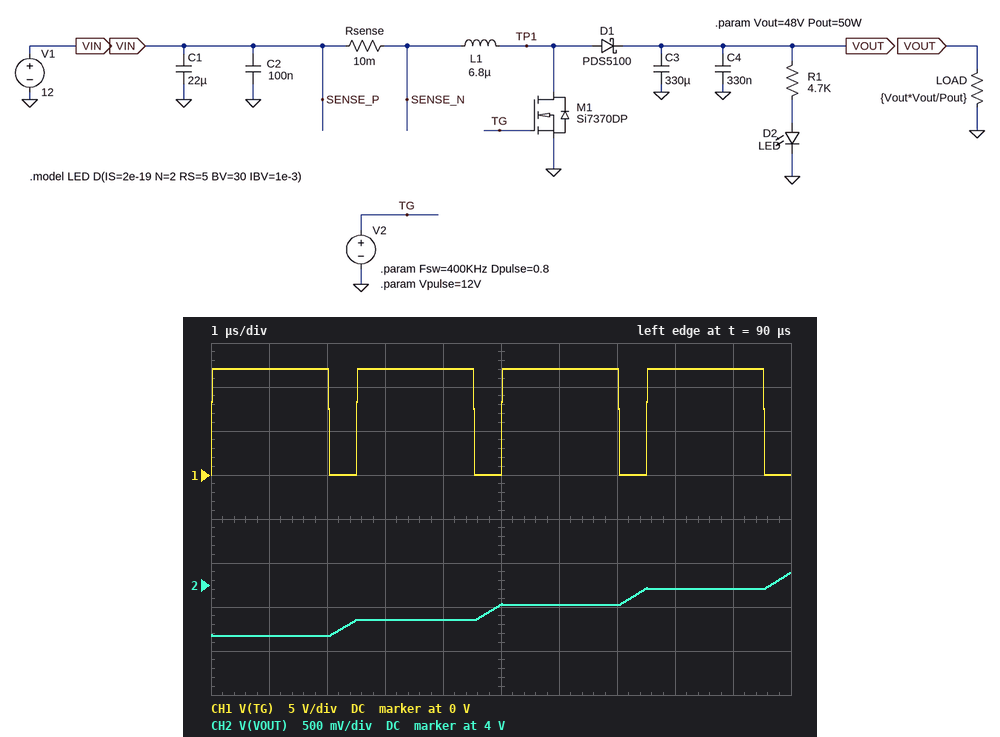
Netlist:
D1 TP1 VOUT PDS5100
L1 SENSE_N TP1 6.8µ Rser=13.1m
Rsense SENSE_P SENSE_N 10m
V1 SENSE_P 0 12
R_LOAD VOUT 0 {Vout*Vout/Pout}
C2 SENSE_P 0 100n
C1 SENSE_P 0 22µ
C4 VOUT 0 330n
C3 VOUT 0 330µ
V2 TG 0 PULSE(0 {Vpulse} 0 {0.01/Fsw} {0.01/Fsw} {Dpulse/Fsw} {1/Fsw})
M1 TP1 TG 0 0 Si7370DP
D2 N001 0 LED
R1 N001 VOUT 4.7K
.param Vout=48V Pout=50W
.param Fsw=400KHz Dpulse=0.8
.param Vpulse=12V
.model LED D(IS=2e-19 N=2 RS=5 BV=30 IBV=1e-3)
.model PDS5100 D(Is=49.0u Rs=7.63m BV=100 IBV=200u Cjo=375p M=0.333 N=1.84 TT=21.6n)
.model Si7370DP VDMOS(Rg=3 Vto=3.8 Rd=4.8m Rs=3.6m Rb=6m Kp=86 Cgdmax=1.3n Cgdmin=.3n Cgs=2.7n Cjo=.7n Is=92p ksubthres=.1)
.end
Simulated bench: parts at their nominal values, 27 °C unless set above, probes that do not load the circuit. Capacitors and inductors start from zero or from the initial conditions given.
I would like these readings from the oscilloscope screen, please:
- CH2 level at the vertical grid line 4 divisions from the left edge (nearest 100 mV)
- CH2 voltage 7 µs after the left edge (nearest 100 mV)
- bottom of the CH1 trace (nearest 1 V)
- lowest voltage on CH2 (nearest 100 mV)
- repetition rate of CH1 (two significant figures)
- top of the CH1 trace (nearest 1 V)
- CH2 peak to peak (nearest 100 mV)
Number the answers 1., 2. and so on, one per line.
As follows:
1. 3.6 V
2. 3.8 V
3. 0 V
4. 3.4 V
5. 400 kHz
6. 12 V
7. 700 mV
